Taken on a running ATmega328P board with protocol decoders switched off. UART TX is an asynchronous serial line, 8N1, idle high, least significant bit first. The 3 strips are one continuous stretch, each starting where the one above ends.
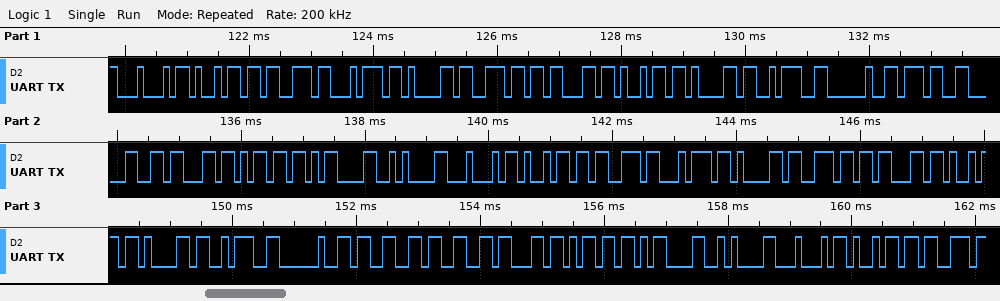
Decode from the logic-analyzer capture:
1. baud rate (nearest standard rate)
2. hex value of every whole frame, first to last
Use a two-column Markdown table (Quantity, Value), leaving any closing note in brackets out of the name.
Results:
| Quantity | Value |
|---|---|
| baud rate | 9600 baud |
| hex value of every whole frame, first to last | 0x44 0x69 0x73 0x74 0x61 0x6E 0x63 0x69 0x61 0x3A 0x20 0x37 0x30 0x63 0x6D 0x0D 0x0A 0x44 0x69 0x73 0x74 0x61 0x6E 0x63 0x69 0x61 0x3A 0x20 0x33 0x33 0x63 0x6D 0x0D 0x0A 0x44 0x69 0x73 |
